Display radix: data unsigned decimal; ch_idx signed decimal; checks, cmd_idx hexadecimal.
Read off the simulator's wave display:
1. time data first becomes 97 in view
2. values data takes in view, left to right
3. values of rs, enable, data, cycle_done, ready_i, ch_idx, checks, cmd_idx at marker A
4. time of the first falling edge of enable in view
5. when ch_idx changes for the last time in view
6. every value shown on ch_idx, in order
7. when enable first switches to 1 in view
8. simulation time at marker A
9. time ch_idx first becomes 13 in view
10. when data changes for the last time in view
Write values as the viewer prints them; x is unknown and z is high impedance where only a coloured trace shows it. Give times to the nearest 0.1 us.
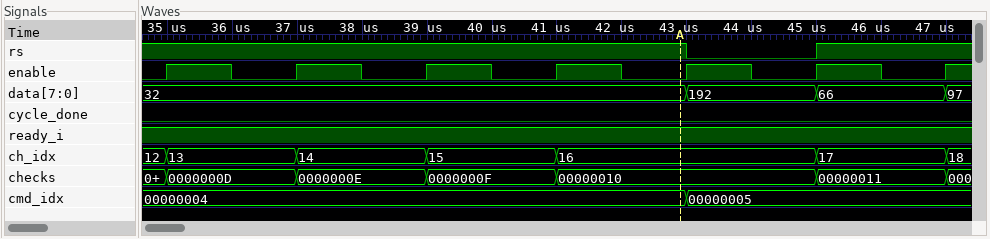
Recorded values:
47 us
32, 192, 66, 97
rs=1, enable=0, data=32, cycle_done=0, ready_i=1, ch_idx=16, checks=00000010, cmd_idx=00000004
36 us
47 us
12, 13, 14, 15, 16, 17, 18
35 us
42.9 us
35 us
47 us
